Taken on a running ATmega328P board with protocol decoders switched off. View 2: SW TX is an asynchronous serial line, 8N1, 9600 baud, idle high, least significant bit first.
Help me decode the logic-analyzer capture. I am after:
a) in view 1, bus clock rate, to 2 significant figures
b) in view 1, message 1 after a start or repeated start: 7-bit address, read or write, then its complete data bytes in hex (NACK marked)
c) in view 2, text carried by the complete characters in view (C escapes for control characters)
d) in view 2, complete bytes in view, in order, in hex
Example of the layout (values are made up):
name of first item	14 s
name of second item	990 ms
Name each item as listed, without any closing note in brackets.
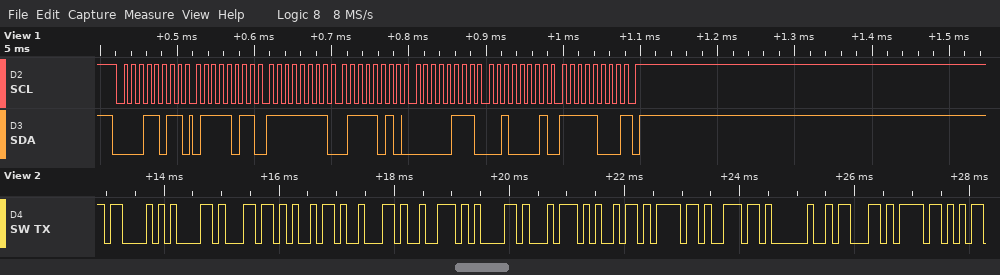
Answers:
in view 1, bus clock rate, to 2 significant figures	100 kHz
in view 1, message 1 after a start or repeated start: 7-bit address, read or write, then its complete data bytes in hex	0x0D read: 7B FF 7A 07 21 F8 NACK
in view 2, text carried by the complete characters in view	"Calibration co"
in view 2, complete bytes in view, in order, in hex	43 61 6C 69 62 72 61 74 69 6F 6E 20 63 6F
